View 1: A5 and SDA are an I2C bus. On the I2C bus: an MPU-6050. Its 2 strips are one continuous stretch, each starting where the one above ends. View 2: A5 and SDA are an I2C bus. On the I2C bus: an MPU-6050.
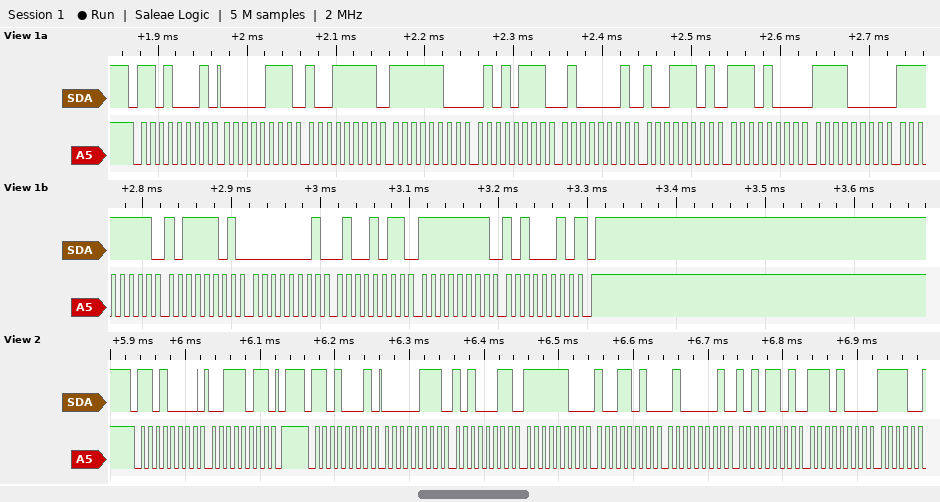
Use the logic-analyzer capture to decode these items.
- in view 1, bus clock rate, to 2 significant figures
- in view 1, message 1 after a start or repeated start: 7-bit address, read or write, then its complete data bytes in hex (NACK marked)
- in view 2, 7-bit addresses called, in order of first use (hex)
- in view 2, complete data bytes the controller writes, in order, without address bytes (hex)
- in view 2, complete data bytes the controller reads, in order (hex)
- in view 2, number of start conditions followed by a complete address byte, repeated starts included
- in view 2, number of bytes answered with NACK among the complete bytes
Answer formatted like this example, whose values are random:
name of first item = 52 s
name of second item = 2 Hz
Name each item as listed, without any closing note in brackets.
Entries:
in view 1, bus clock rate, to 2 significant figures = 100 kHz
in view 1, message 1 after a start or repeated start: 7-bit address, read or write, then its complete data bytes in hex = 0x68 read: 07 9F FC 57 41 9D E8 F0 FF BD 01 4B FF A2 NACK
in view 2, 7-bit addresses called, in order of first use = 0x68
in view 2, complete data bytes the controller writes, in order, without address bytes = 3B
in view 2, complete data bytes the controller reads, in order = 07 A3 FC 9A 41 AD E8
in view 2, number of start conditions followed by a complete address byte, repeated starts included = 2
in view 2, number of bytes answered with NACK among the complete bytes = 0
